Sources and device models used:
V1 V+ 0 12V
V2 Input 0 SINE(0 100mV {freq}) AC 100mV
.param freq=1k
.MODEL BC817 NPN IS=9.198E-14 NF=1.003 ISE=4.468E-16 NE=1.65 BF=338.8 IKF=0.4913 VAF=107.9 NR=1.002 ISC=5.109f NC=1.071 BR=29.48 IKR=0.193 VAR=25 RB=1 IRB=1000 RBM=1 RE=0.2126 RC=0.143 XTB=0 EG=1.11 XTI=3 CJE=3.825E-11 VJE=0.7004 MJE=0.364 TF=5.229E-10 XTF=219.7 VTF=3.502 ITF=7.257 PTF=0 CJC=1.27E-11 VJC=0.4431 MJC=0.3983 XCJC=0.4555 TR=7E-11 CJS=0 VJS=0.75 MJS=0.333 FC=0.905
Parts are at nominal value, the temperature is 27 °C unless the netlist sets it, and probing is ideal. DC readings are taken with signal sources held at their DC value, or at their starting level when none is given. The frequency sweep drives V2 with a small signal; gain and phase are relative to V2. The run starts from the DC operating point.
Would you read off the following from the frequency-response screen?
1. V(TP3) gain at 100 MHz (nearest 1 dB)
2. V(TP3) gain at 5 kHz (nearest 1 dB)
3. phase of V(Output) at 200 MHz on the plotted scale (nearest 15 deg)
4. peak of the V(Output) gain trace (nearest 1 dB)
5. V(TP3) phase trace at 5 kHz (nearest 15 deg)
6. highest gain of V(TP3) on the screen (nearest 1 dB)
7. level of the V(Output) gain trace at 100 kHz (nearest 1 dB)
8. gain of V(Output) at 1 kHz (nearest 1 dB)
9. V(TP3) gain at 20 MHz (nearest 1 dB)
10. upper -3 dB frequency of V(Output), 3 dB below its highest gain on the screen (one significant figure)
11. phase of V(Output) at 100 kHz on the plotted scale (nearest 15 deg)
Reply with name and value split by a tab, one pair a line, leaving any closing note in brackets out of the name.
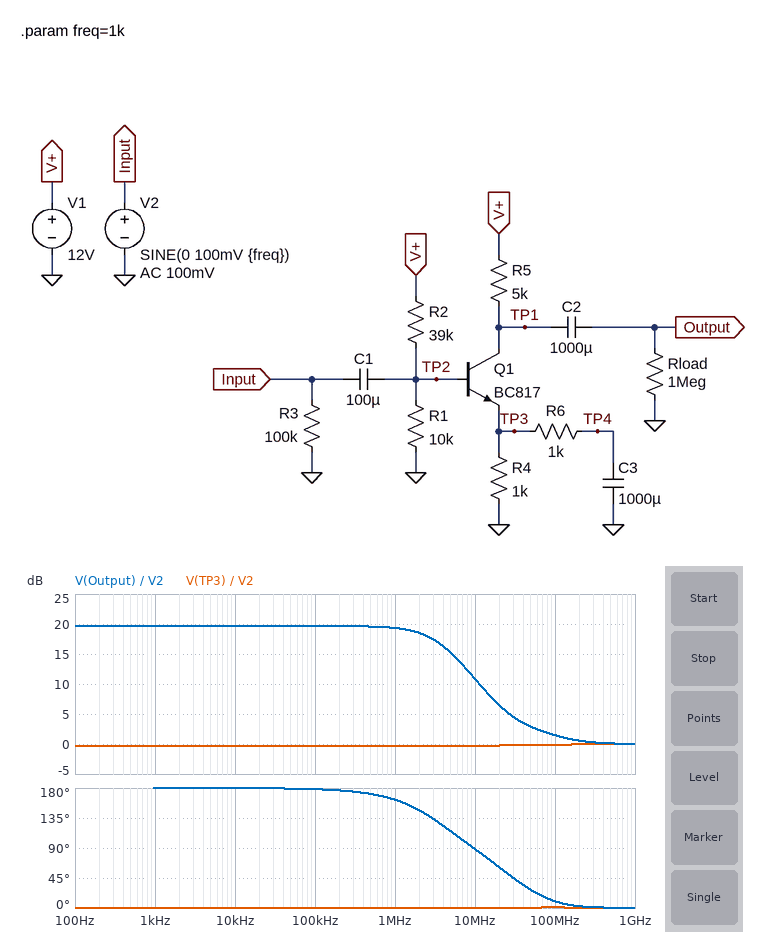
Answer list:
V(TP3) gain at 100 MHz	0 dB
V(TP3) gain at 5 kHz	0 dB
phase of V(Output) at 200 MHz on the plotted scale	0 deg
peak of the V(Output) gain trace	20 dB
V(TP3) phase trace at 5 kHz	0 deg
highest gain of V(TP3) on the screen	0 dB
level of the V(Output) gain trace at 100 kHz	20 dB
gain of V(Output) at 1 kHz	20 dB
V(TP3) gain at 20 MHz	0 dB
upper -3 dB frequency of V(Output), 3 dB below its highest gain on the screen	4 MHz
phase of V(Output) at 100 kHz on the plotted scale	180 deg
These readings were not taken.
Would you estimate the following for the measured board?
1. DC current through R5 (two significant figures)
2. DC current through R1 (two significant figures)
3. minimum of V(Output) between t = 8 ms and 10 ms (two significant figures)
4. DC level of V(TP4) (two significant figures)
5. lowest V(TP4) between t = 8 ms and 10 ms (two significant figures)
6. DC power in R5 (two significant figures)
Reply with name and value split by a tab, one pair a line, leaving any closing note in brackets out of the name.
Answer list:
DC current through R5	1.8 mA
DC current through R1	240 µA
minimum of V(Output) between t = 8 ms and 10 ms	-960 mV
DC level of V(TP4)	1.8 V
lowest V(TP4) between t = 8 ms and 10 ms	1.8 V
DC power in R5	16 mW
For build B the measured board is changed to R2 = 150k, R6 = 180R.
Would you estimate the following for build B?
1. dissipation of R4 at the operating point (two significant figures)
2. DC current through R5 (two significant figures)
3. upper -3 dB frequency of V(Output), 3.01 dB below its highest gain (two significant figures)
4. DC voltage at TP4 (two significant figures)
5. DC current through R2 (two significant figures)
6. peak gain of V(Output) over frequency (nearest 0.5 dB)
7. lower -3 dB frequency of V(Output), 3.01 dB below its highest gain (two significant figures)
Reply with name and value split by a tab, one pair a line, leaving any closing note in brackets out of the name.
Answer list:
dissipation of R4 at the operating point	36 µW
DC current through R5	190 µA
upper -3 dB frequency of V(Output), 3.01 dB below its highest gain	8.6 MHz
DC voltage at TP4	190 mV
DC current through R2	75 µA
peak gain of V(Output) over frequency	24.5 dB
lower -3 dB frequency of V(Output), 3.01 dB below its highest gain	560 mHz
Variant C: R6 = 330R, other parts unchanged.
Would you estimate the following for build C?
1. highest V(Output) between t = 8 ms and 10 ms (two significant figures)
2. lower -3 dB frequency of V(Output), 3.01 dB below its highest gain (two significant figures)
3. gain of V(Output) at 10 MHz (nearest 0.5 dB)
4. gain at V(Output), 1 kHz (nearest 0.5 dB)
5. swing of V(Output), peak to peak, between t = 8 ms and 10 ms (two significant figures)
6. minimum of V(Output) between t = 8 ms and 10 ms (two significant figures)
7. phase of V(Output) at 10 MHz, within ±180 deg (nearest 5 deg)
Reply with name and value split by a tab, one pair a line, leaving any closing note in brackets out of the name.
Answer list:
highest V(Output) between t = 8 ms and 10 ms	1.9 V
lower -3 dB frequency of V(Output), 3.01 dB below its highest gain	530 mHz
gain of V(Output) at 10 MHz	16.5 dB
gain at V(Output), 1 kHz	25.5 dB
swing of V(Output), peak to peak, between t = 8 ms and 10 ms	3.1 V
minimum of V(Output) between t = 8 ms and 10 ms	-1.2 V
phase of V(Output) at 10 MHz, within ±180 deg	95 deg
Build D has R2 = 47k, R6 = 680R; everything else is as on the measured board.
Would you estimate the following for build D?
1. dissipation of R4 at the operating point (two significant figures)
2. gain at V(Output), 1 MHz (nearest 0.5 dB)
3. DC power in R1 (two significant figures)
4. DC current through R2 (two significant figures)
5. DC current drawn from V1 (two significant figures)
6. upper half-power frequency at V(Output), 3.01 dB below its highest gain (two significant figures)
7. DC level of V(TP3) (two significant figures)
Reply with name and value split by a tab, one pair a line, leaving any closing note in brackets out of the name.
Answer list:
dissipation of R4 at the operating point	2.1 mW
gain at V(Output), 1 MHz	21.0 dB
DC power in R1	430 µW
DC current through R2	210 µA
DC current drawn from V1	1.7 mA
upper half-power frequency at V(Output), 3.01 dB below its highest gain	5.5 MHz
DC level of V(TP3)	1.5 V
